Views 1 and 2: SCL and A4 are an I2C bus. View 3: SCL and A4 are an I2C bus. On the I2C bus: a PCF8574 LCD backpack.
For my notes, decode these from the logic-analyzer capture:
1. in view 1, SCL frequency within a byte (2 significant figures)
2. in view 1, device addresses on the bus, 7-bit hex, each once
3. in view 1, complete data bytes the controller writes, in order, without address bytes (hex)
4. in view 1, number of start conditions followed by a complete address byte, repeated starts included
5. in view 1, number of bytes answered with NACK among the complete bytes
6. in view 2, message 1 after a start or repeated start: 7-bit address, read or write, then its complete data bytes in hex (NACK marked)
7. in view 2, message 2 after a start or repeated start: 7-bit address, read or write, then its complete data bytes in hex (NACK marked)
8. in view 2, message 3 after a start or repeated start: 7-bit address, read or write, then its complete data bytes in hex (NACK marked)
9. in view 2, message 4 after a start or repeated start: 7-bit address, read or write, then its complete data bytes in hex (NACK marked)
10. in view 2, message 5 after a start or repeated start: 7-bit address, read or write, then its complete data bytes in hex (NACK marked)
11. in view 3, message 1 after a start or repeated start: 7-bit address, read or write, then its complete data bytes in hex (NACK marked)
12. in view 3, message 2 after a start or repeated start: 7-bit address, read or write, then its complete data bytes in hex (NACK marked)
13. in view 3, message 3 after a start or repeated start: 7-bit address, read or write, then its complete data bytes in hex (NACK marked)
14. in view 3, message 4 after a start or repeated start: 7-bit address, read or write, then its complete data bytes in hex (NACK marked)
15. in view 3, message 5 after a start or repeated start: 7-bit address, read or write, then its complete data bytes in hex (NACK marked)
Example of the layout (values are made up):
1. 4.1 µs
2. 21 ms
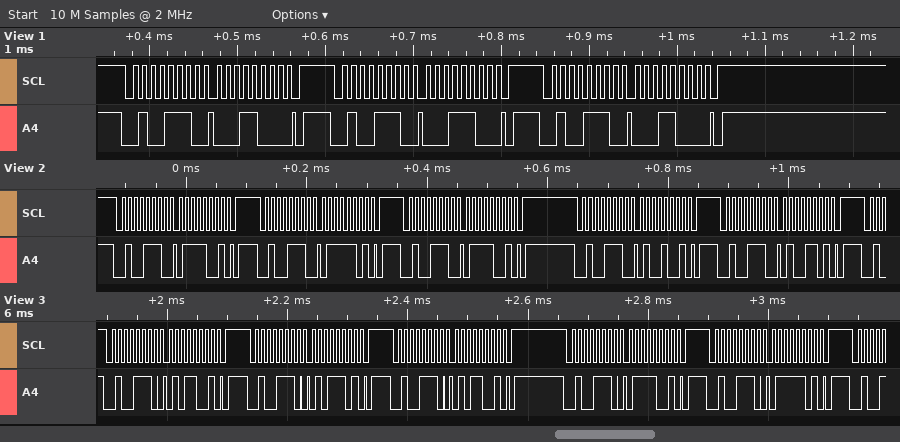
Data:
1. 100 kHz
2. 0x27
3. 18 1C 18
4. 3
5. 0
6. 0x27 write: 79
7. 0x27 write: 7D
8. 0x27 write: 79
9. 0x27 write: 49
10. 0x27 write: 4D
11. 0x27 write: 59
12. 0x27 write: 5D
13. 0x27 write: 59
14. 0x27 write: 79
15. 0x27 write: 7D
